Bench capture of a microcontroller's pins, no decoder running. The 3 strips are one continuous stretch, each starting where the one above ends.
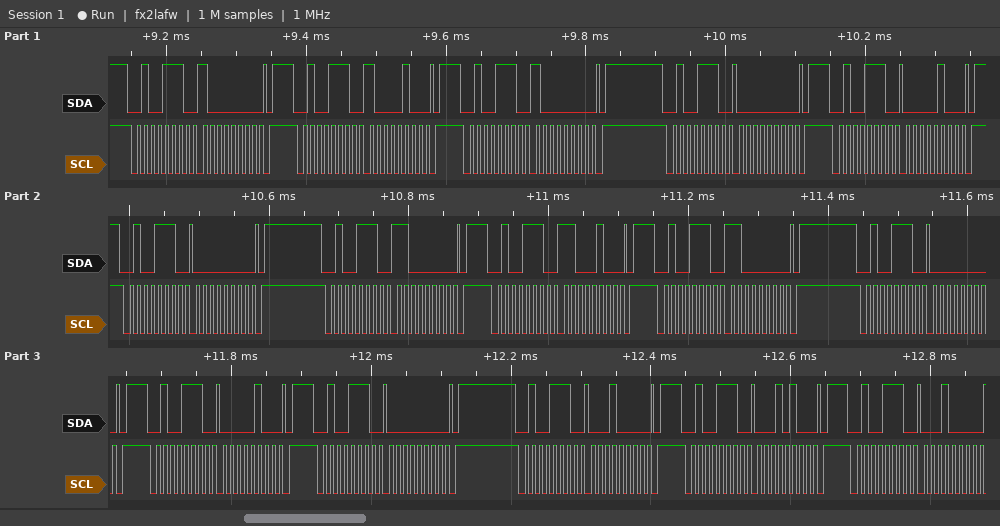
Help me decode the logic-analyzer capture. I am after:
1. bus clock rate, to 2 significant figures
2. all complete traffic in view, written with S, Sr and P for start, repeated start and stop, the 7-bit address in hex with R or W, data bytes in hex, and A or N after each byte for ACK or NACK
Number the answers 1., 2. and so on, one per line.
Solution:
1. 100 kHz
2. S 27W A 80 A P S 27W A 84 A P S 27W A 80 A P S 27W A 00 A P S 27W A 04 A P S 27W A 00 A P S 27W A C0 A P S 27W A C4 A P S 27W A C0 A P S 27W A 00 A P S 27W A 04 A P S 27W A 00 A P S 27W A 10 A P S 27W A 14 A P S 27W A 10 A
